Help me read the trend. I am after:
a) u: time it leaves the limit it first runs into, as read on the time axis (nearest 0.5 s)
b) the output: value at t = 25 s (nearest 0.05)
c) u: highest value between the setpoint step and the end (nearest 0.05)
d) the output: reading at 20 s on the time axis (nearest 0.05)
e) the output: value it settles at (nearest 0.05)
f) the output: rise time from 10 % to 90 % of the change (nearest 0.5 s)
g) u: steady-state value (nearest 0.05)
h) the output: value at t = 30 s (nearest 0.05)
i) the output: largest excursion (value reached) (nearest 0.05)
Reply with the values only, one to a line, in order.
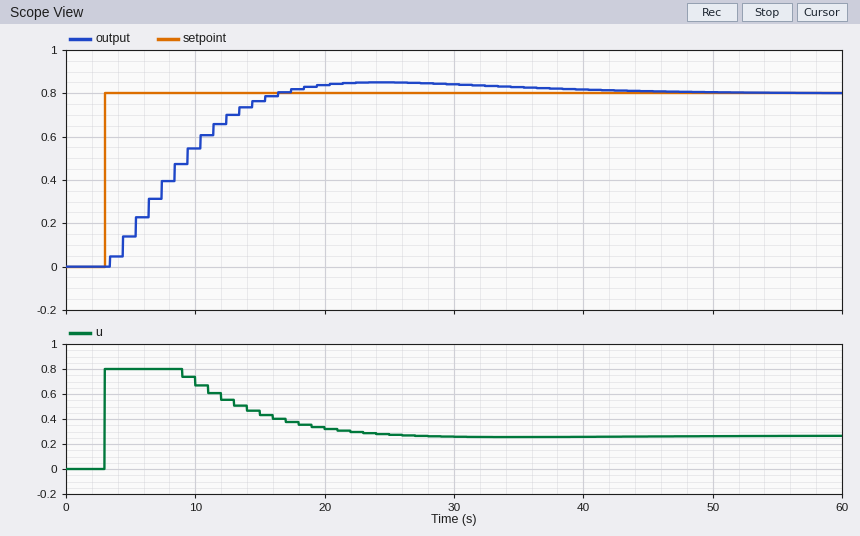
9.0 s
0.85
0.80
0.85
0.80
9.0 s
0.25
0.85
0.85
